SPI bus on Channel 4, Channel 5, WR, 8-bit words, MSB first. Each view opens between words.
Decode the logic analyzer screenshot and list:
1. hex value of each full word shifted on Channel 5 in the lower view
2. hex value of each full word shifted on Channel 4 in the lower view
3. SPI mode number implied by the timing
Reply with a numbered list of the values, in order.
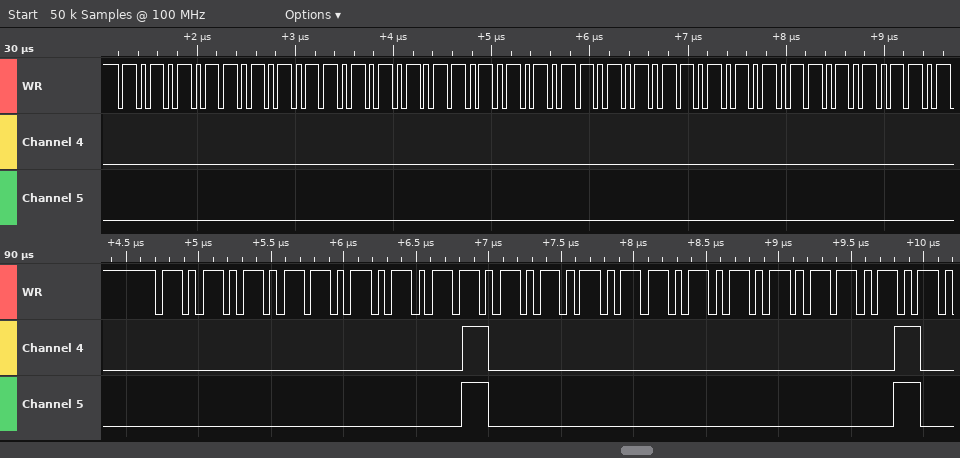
1. 00, 01, 00, 00
2. 00, 01, 00, 00
3. 2
